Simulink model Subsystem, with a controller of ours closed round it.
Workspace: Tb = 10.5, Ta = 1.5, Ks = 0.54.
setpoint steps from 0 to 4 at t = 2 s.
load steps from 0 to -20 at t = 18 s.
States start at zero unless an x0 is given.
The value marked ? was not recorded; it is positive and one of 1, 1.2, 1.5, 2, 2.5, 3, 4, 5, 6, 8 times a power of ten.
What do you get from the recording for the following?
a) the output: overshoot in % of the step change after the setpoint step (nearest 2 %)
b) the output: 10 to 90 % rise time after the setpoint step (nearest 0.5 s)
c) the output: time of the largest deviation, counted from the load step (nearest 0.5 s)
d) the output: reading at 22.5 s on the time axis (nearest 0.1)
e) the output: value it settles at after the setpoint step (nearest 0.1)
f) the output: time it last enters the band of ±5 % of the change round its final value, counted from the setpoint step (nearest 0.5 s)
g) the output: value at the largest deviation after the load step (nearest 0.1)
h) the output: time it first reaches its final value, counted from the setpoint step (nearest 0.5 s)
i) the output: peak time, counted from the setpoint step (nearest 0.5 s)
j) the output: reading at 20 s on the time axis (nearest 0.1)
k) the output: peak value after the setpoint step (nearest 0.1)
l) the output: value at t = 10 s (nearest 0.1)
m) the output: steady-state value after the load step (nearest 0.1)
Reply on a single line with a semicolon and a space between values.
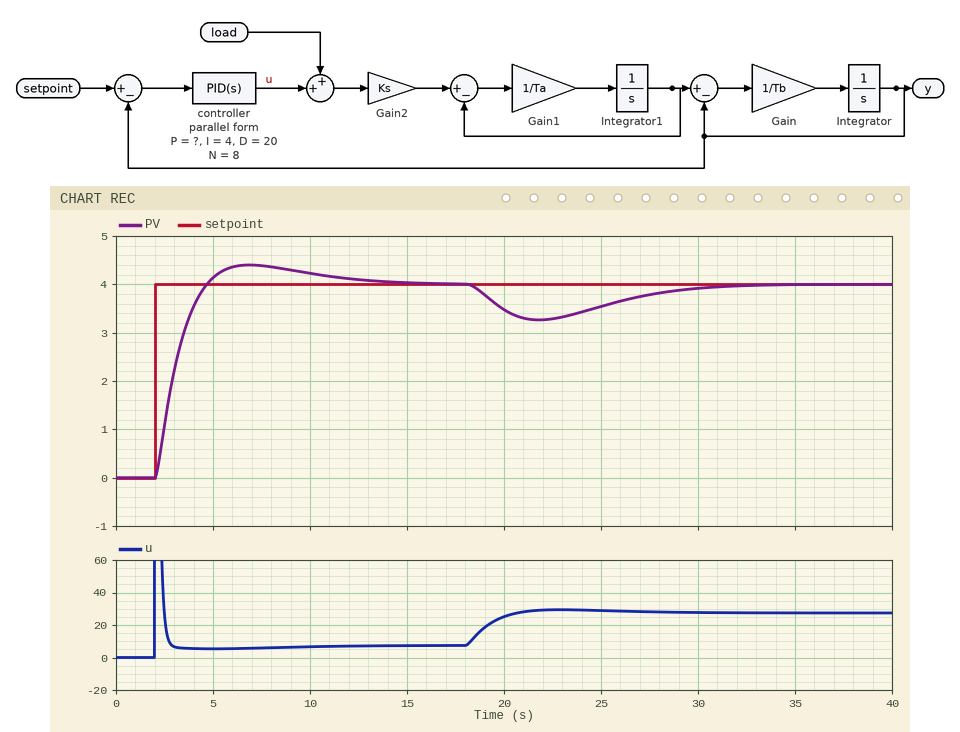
10 %; 2.0 s; 4.0 s; 3.3; 4.0; 8.5 s; 3.3; 2.5 s; 5.0 s; 3.5; 4.4; 4.2; 4.0
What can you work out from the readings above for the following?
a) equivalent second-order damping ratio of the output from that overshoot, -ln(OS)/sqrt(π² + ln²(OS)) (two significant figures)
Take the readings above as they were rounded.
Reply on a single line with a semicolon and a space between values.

0.59
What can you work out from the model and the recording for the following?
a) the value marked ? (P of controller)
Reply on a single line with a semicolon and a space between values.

20
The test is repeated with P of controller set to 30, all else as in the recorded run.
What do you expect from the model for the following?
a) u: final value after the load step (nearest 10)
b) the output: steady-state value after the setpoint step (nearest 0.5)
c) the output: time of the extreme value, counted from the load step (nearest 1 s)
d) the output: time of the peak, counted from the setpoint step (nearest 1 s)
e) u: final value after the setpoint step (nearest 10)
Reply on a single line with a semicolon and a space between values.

30; 4.0; 3 s; 3 s; 10
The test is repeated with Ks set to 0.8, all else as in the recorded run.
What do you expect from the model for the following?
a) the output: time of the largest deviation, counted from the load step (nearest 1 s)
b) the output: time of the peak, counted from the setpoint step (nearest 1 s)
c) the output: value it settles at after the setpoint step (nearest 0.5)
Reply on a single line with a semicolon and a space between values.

3 s; 4 s; 4.0
